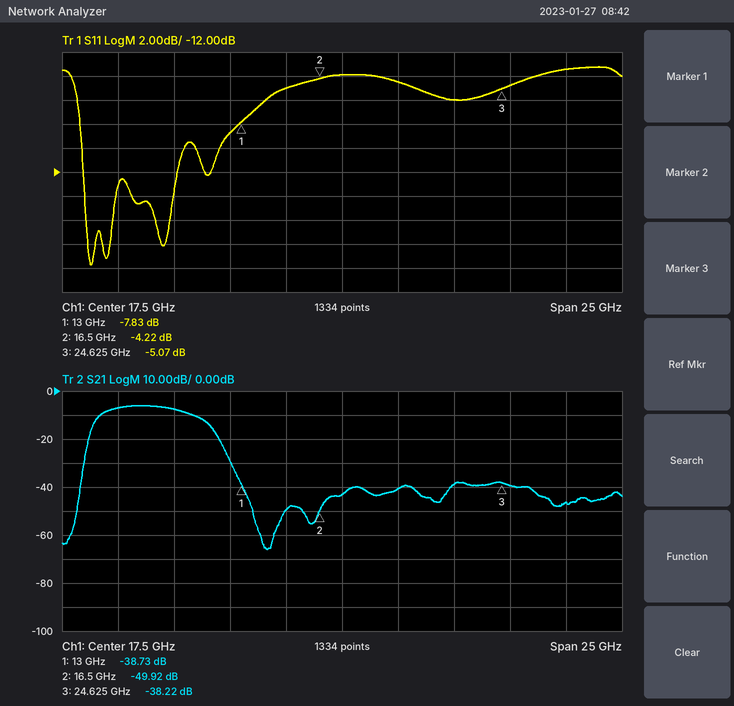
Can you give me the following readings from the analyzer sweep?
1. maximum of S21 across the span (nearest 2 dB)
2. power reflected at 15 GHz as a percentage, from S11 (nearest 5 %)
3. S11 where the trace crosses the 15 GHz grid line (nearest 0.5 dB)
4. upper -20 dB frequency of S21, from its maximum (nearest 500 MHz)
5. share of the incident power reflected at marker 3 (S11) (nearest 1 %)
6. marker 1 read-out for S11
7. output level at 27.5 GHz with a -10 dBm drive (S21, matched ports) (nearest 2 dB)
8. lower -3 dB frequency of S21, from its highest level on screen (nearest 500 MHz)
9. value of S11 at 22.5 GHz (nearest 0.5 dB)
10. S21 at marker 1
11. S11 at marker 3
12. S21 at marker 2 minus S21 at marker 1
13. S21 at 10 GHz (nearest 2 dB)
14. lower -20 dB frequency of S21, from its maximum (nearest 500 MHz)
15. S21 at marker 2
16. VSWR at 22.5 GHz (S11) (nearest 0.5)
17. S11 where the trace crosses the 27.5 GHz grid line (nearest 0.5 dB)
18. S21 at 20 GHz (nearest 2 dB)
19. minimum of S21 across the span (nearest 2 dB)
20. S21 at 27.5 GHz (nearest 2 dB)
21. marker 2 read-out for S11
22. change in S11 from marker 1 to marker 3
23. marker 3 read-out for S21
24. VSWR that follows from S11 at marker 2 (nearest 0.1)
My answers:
-6 dB
30 %
-5.0 dB
12.5 GHz
31 %
-7.83 dB
-56 dBm
7.0 GHz
-6.0 dB
-38.73 dB
-5.07 dB
-11.19 dB
-8 dB
6.0 GHz
-49.92 dB
3.0
-3.5 dB
-40 dB
-66 dB
-46 dB
-4.22 dB
2.76 dB
-38.22 dB
4.2
